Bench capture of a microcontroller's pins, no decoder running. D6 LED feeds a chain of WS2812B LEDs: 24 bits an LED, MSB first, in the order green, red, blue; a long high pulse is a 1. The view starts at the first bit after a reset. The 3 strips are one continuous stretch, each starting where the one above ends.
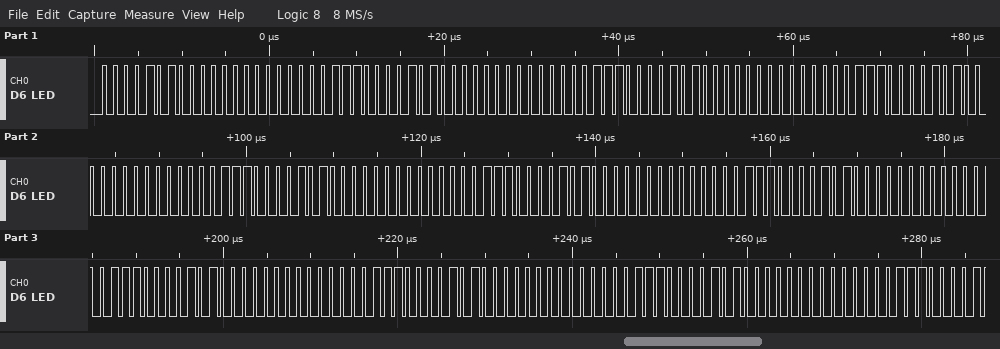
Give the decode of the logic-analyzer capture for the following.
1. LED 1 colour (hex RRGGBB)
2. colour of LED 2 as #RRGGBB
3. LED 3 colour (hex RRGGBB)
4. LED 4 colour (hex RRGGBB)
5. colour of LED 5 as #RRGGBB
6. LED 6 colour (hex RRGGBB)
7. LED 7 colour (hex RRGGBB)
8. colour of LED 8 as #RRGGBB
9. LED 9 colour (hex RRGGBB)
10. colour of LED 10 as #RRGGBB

#000A07
#000A07
#000A07
#000A07
#000A07
#000A07
#000A07
#000A07
#000A07
#000A07
